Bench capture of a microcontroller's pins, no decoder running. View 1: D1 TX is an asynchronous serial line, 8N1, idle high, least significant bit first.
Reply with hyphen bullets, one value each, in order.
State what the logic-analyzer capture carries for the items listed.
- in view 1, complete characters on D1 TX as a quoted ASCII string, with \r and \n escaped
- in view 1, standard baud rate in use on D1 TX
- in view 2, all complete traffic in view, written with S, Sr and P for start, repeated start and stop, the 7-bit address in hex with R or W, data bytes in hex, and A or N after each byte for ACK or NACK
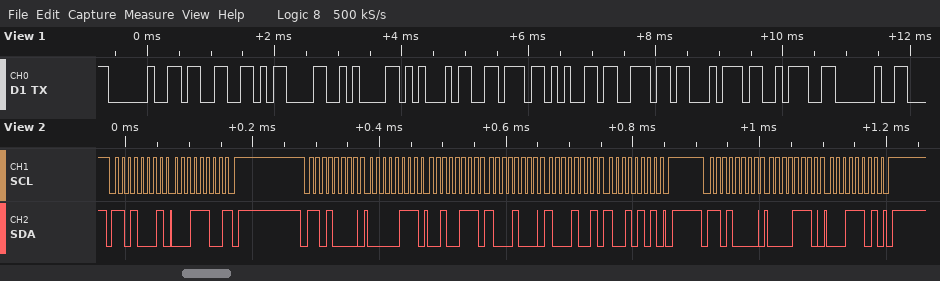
- " 3\r\nEvent: "
- 9600 baud
- S 68R A 1C N P S 68W A 07 A 27 A 88 A 89 A 95 A P S 68W A 0E A 1D A P
